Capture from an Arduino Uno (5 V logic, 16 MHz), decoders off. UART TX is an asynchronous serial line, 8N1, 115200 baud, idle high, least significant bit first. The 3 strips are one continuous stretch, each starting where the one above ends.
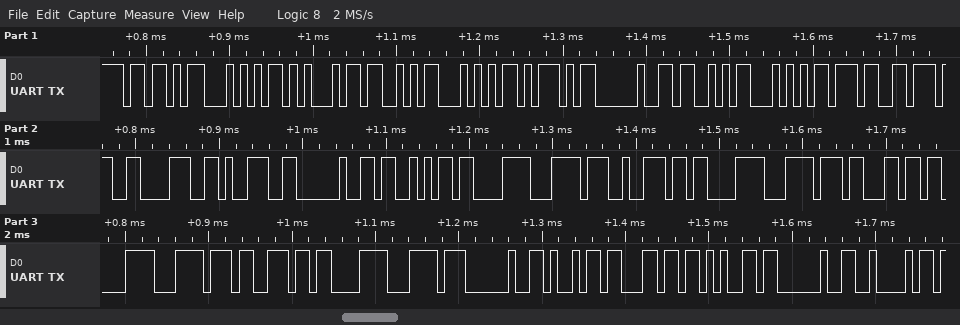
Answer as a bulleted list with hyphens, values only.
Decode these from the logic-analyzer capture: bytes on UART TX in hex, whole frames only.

- 5B 54 45 53 54 5D 20 53 54 37 37 38 39 20 53 C3 BC 72 C3 BC 63 C3 BC 73 C3 BC 20 69 6C 65 20 42
